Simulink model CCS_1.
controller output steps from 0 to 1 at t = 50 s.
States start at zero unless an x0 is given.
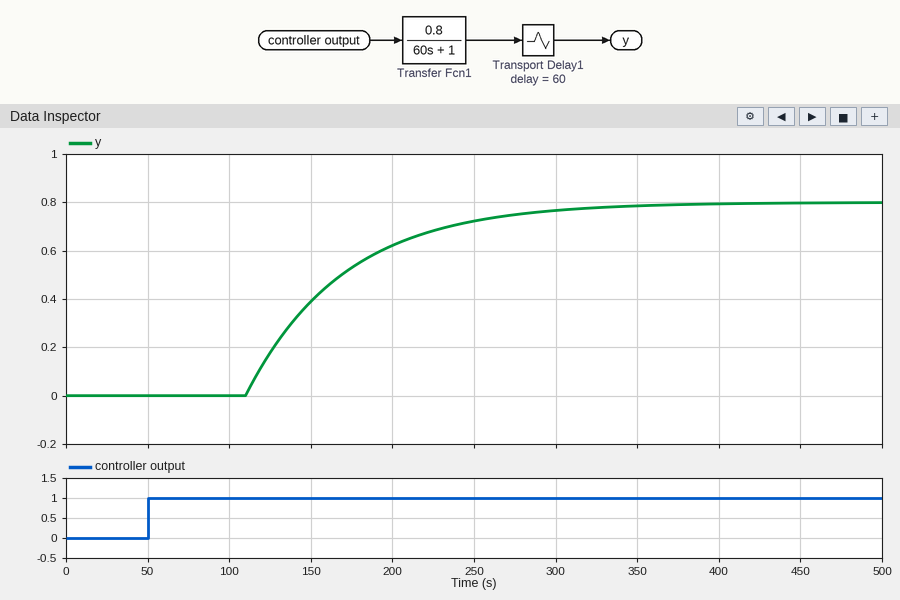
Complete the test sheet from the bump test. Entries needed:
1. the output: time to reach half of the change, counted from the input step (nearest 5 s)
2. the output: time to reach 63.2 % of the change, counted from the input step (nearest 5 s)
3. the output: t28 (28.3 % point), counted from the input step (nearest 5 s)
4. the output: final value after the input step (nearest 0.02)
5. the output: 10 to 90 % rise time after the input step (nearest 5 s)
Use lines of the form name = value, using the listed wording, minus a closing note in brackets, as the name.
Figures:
the output: time to reach half of the change, counted from the input step = 100 s
the output: time to reach 63.2 % of the change, counted from the input step = 120 s
the output: t28 (28.3 % point), counted from the input step = 80 s
the output: final value after the input step = 0.80
the output: 10 to 90 % rise time after the input step = 130 s
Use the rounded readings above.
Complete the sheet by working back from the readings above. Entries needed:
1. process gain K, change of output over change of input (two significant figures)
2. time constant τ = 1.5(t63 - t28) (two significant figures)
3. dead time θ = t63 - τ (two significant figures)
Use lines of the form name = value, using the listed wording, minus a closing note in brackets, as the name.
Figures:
process gain K, change of output over change of input = 0.80
time constant τ = 1.5(t63 - t28) = 60 s
dead time θ = t63 - τ = 60 s
